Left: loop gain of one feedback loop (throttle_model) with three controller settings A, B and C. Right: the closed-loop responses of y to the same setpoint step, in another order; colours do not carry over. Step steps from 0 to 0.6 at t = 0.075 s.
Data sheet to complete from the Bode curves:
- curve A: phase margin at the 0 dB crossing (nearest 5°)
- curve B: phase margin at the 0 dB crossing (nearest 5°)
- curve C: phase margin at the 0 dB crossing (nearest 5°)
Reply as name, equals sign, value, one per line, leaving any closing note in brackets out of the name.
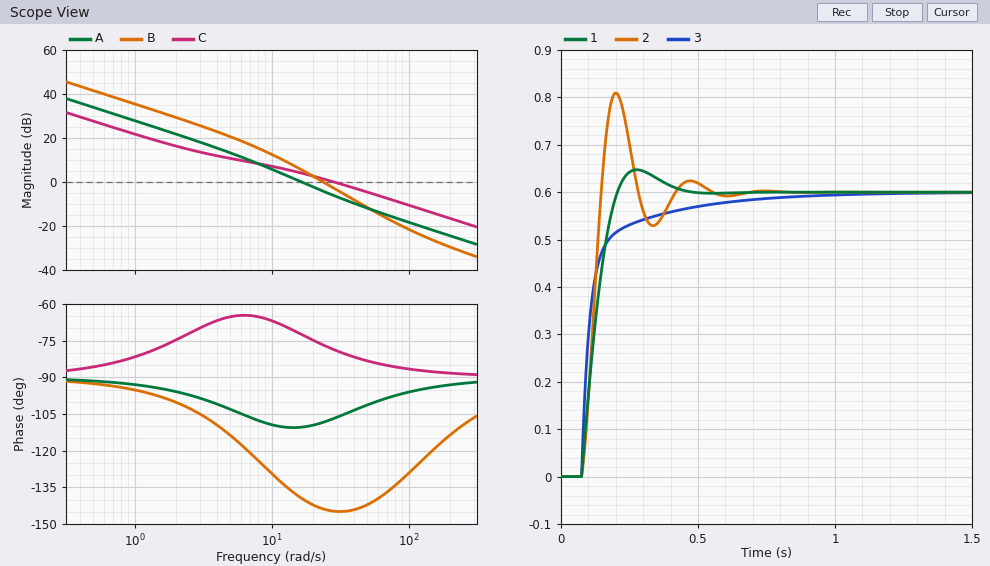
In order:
curve A: phase margin at the 0 dB crossing = 70°
curve B: phase margin at the 0 dB crossing = 35°
curve C: phase margin at the 0 dB crossing = 100°
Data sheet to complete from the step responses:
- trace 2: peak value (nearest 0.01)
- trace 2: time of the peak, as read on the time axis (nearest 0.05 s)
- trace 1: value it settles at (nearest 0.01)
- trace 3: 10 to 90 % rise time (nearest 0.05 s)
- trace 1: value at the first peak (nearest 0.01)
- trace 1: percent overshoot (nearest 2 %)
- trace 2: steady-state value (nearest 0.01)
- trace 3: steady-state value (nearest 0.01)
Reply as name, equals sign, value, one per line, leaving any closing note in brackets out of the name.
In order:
trace 2: peak value = 0.81
trace 2: time of the peak, as read on the time axis = 0.20 s
trace 1: value it settles at = 0.60
trace 3: 10 to 90 % rise time = 0.20 s
trace 1: value at the first peak = 0.65
trace 1: percent overshoot = 8 %
trace 2: steady-state value = 0.60
trace 3: steady-state value = 0.60
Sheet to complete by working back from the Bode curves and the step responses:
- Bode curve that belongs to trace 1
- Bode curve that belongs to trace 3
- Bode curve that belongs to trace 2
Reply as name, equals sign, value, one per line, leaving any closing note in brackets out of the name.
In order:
Bode curve that belongs to trace 1 = A
Bode curve that belongs to trace 3 = C
Bode curve that belongs to trace 2 = B
